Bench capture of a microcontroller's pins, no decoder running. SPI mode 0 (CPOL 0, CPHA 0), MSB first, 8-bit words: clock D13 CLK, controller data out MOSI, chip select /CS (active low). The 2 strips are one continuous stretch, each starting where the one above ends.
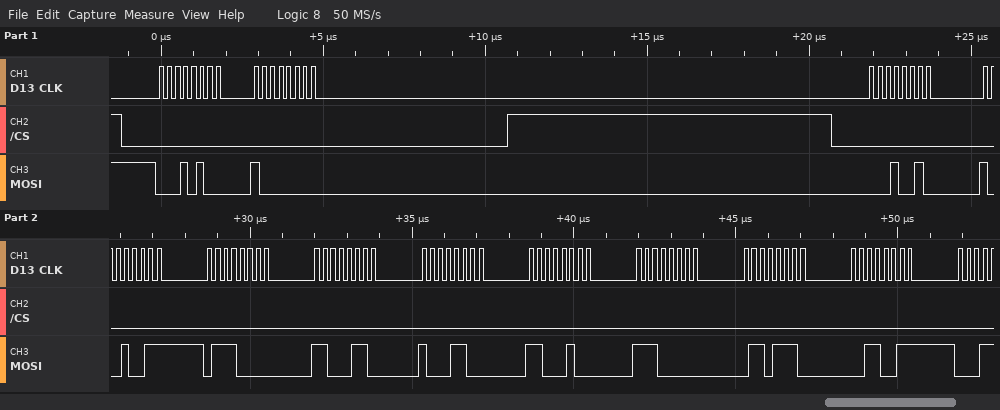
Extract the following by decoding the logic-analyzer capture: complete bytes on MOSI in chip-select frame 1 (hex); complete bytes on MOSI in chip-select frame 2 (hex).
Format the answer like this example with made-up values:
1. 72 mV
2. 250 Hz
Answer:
1. 14 80
2. 12 93 70 C6 8C C4 E0 6E 33
